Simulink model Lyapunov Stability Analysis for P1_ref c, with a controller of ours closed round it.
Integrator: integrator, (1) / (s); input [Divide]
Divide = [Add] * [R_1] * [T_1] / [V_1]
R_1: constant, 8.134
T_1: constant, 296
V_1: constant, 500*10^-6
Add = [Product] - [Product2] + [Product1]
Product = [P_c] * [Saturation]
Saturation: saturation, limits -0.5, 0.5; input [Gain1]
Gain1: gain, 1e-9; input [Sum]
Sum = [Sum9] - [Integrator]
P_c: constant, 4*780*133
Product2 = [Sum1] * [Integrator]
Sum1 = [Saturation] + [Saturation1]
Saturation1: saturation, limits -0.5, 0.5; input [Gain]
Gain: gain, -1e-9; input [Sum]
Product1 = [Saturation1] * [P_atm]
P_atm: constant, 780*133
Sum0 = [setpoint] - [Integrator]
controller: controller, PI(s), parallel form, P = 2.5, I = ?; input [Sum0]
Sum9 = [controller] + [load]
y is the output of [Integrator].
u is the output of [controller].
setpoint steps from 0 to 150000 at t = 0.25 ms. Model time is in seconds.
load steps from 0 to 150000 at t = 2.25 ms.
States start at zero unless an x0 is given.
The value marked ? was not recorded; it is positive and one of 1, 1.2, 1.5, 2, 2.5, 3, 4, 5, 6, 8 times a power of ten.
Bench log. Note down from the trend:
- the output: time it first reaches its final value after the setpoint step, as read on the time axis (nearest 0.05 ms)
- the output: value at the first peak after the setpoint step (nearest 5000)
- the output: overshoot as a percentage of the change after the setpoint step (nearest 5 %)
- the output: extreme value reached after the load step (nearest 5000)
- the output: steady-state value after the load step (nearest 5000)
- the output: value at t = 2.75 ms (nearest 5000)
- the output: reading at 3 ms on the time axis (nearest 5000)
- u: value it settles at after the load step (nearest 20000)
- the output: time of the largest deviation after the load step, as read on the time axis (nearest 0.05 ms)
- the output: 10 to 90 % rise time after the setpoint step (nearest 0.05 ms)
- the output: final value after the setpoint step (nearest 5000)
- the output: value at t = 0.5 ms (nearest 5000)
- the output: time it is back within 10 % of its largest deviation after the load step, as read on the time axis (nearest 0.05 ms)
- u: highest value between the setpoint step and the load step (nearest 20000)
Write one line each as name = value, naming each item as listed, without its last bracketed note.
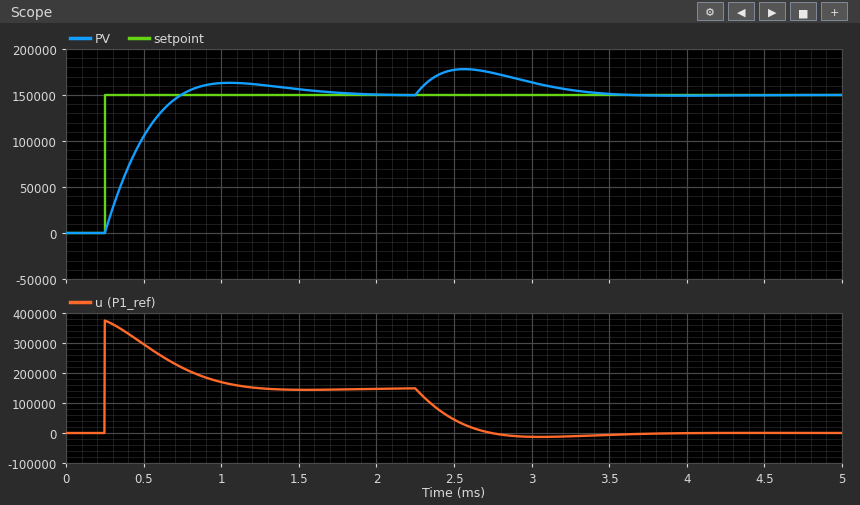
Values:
the output: time it first reaches its final value after the setpoint step, as read on the time axis = 0.75 ms
the output: value at the first peak after the setpoint step = 165000
the output: overshoot as a percentage of the change after the setpoint step = 10 %
the output: extreme value reached after the load step = 180000
the output: steady-state value after the load step = 150000
the output: value at t = 2.75 ms = 175000
the output: reading at 3 ms on the time axis = 165000
u: value it settles at after the load step = 0
the output: time of the largest deviation after the load step, as read on the time axis = 2.55 ms
the output: 10 to 90 % rise time after the setpoint step = 0.35 ms
the output: final value after the setpoint step = 150000
the output: value at t = 0.5 ms = 105000
the output: time it is back within 10 % of its largest deviation after the load step, as read on the time axis = 3.40 ms
u: highest value between the setpoint step and the load step = 380000
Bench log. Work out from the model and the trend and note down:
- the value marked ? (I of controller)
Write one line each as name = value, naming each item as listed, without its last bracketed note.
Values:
the value marked ? = 8000
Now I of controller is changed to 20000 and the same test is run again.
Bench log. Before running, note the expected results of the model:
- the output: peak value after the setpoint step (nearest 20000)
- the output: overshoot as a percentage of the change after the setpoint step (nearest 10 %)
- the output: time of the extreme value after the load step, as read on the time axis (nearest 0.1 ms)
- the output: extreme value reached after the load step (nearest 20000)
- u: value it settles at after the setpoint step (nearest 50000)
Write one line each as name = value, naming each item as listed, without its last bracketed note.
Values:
the output: peak value after the setpoint step = 180000
the output: overshoot as a percentage of the change after the setpoint step = 20 %
the output: time of the extreme value after the load step, as read on the time axis = 2.5 ms
the output: extreme value reached after the load step = 180000
u: value it settles at after the setpoint step = 150000
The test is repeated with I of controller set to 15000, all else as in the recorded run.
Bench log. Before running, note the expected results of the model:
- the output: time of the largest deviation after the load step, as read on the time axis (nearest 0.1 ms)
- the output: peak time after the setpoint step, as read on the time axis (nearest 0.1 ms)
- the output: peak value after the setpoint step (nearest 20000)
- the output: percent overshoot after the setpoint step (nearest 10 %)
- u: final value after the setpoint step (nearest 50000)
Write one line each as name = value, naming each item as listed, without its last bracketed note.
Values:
the output: time of the largest deviation after the load step, as read on the time axis = 2.5 ms
the output: peak time after the setpoint step, as read on the time axis = 0.8 ms
the output: peak value after the setpoint step = 180000
the output: percent overshoot after the setpoint step = 20 %
u: final value after the setpoint step = 150000
